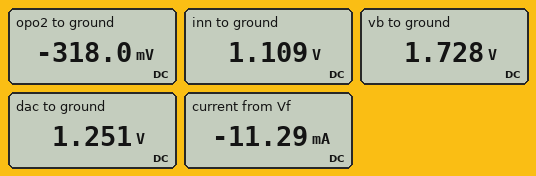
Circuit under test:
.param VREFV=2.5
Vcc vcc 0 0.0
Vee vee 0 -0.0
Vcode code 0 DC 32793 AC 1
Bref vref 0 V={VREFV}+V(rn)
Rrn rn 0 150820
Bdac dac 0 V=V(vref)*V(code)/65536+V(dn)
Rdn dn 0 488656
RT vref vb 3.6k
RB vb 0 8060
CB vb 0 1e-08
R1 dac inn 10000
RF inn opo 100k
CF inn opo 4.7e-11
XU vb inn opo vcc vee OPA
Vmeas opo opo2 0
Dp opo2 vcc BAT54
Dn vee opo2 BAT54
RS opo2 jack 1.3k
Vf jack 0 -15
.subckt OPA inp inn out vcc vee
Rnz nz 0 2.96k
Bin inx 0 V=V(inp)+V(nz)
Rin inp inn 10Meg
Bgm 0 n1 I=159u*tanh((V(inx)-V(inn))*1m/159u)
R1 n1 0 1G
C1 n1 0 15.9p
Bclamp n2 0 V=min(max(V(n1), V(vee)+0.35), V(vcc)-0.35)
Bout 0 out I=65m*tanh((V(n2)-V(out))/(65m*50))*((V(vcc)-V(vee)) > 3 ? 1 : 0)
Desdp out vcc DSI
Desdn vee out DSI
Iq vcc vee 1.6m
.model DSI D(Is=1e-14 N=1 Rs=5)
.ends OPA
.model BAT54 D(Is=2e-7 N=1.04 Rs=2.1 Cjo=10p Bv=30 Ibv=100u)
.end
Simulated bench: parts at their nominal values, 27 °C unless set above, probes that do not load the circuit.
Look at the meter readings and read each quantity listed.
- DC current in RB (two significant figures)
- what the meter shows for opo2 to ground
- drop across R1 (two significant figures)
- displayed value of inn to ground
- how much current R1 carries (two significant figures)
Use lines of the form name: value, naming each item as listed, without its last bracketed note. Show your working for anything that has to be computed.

DC current in RB: (1.728 V) / 8.06 kΩ = 210 µA
what the meter shows for opo2 to ground: -318.0 mV
drop across R1: 1.251 V - 1.109 V = 140 mV
displayed value of inn to ground: 1.109 V
how much current R1 carries: (1.251 V - 1.109 V) / 10 kΩ = 14 µA
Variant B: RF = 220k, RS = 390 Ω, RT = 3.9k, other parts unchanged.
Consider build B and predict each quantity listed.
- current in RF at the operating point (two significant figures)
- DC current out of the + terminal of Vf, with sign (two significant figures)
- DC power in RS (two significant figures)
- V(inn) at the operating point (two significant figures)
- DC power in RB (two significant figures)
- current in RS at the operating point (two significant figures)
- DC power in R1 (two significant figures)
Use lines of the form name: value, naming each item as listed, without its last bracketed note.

current in RF at the operating point: 7.2 µA
DC current out of the + terminal of Vf, with sign: -37 mA
DC power in RS: 550 mW
V(inn) at the operating point: 1.2 V
DC power in RB: 350 µW
current in RS at the operating point: 37 mA
DC power in R1: 510 nW
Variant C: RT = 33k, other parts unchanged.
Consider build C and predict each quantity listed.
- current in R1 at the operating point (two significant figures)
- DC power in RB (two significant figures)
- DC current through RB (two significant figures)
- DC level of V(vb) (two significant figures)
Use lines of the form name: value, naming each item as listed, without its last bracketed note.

current in R1 at the operating point: 14 µA
DC power in RB: 30 µW
DC current through RB: 61 µA
DC level of V(vb): 490 mV
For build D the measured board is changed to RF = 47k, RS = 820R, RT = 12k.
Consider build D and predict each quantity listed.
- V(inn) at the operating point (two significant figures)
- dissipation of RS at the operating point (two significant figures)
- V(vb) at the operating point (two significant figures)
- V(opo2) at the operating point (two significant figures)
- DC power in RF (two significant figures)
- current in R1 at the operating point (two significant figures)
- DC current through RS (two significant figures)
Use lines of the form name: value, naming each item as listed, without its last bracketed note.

V(inn) at the operating point: 970 mV
dissipation of RS at the operating point: 260 mW
V(vb) at the operating point: 1.0 V
V(opo2) at the operating point: -340 mV
DC power in RF: 37 µW
current in R1 at the operating point: 28 µA
DC current through RS: 18 mA
